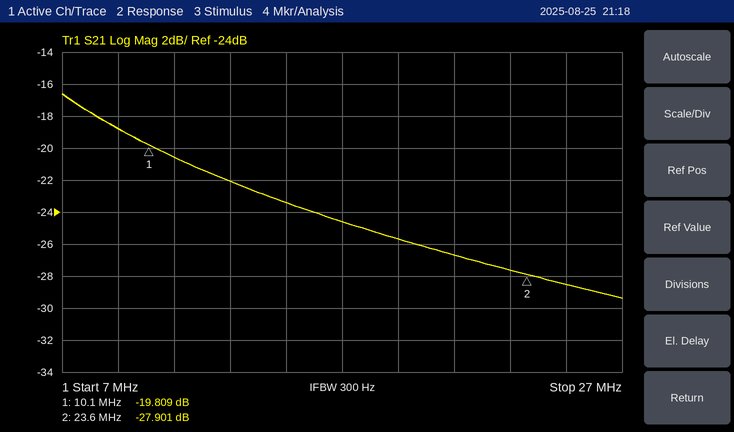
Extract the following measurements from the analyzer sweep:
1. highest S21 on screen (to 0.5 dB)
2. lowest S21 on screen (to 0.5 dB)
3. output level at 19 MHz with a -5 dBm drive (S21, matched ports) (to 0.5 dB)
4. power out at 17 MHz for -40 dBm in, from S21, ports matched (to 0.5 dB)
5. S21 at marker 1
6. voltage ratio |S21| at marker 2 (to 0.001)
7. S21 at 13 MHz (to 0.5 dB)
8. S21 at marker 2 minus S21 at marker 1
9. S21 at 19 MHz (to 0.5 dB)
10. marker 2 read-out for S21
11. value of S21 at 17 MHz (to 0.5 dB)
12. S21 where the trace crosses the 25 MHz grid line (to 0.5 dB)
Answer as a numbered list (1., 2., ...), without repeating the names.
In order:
1. -16.5 dB
2. -29.5 dB
3. -30.5 dBm
4. -64.5 dBm
5. -19.809 dB
6. 0.040
7. -22.0 dB
8. -8.092 dB
9. -25.5 dB
10. -27.901 dB
11. -24.5 dB
12. -28.5 dB
